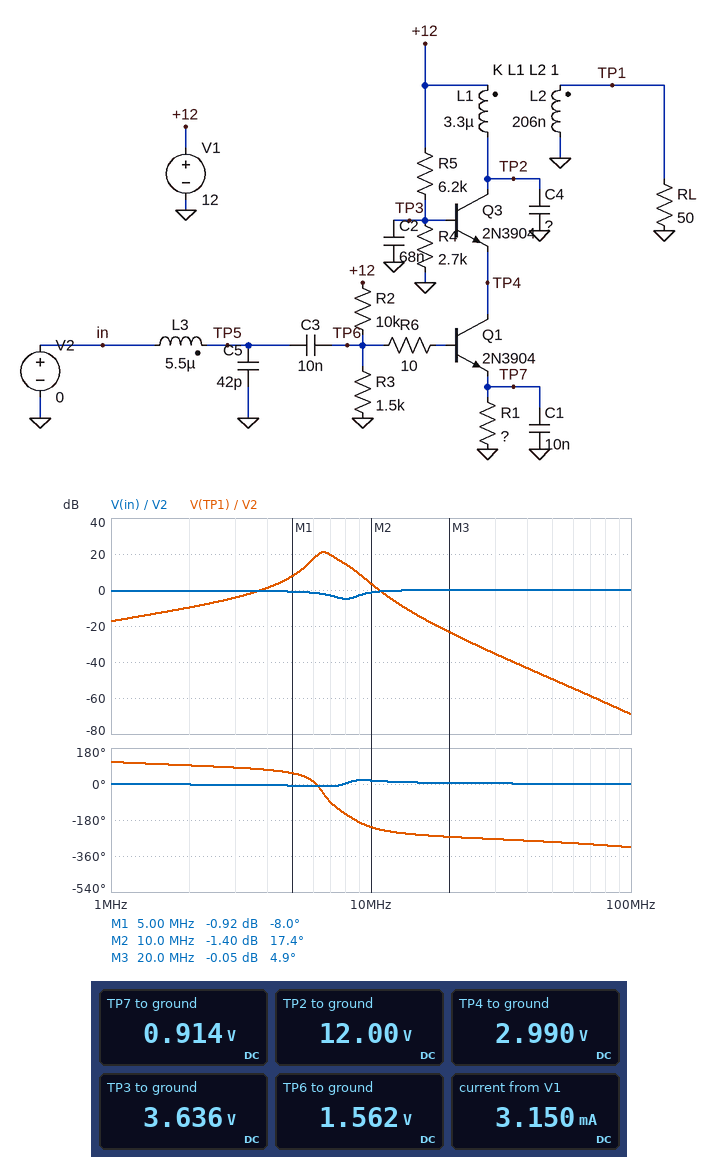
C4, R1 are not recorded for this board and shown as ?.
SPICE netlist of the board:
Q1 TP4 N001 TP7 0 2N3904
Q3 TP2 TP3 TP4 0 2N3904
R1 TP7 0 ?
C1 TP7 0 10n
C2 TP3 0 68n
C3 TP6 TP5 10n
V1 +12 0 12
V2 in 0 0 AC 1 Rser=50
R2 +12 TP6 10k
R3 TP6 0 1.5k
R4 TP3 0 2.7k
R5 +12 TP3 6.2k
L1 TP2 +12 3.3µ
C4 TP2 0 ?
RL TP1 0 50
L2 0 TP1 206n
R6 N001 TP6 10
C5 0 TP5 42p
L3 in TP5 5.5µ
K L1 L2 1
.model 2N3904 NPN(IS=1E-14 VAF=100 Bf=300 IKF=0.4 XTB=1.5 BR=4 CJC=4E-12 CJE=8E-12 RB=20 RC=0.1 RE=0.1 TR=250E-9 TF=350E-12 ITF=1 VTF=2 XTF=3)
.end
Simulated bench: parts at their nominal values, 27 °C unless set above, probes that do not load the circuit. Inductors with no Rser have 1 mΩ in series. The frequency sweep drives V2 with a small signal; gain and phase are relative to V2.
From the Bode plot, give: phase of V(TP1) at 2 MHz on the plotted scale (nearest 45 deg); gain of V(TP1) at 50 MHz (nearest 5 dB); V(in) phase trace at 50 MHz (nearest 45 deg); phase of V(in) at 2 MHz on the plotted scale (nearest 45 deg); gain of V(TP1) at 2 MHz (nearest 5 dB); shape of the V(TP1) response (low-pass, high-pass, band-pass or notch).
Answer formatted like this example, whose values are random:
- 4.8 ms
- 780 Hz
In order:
- 90 deg
- -50 dB
- 0 deg
- 0 deg
- -10 dB
- band-pass
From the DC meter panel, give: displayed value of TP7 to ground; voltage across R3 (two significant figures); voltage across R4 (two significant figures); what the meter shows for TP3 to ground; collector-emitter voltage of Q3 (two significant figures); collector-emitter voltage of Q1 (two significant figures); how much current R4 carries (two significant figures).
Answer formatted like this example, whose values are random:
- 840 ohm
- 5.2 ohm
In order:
- 0.914 V
- 1.6 V
- 3.6 V
- 3.636 V
- 9.0 V
- 2.1 V
- 1.3 mA
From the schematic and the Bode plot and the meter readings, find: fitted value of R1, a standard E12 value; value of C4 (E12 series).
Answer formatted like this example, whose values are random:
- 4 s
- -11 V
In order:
- 1.2 kΩ
- 180 pF
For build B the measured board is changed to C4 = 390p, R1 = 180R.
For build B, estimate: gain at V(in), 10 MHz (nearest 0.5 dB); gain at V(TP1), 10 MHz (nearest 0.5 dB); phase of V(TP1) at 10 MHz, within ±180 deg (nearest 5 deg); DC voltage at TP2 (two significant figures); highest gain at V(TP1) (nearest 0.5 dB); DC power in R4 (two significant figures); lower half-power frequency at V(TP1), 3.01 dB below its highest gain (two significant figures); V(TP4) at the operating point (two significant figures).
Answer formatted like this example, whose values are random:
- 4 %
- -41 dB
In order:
- -0.5 dB
- 2.0 dB
- 120 deg
- 12 V
- 34.0 dB
- 4.8 mW
- 4.2 MHz
- 2.9 V
